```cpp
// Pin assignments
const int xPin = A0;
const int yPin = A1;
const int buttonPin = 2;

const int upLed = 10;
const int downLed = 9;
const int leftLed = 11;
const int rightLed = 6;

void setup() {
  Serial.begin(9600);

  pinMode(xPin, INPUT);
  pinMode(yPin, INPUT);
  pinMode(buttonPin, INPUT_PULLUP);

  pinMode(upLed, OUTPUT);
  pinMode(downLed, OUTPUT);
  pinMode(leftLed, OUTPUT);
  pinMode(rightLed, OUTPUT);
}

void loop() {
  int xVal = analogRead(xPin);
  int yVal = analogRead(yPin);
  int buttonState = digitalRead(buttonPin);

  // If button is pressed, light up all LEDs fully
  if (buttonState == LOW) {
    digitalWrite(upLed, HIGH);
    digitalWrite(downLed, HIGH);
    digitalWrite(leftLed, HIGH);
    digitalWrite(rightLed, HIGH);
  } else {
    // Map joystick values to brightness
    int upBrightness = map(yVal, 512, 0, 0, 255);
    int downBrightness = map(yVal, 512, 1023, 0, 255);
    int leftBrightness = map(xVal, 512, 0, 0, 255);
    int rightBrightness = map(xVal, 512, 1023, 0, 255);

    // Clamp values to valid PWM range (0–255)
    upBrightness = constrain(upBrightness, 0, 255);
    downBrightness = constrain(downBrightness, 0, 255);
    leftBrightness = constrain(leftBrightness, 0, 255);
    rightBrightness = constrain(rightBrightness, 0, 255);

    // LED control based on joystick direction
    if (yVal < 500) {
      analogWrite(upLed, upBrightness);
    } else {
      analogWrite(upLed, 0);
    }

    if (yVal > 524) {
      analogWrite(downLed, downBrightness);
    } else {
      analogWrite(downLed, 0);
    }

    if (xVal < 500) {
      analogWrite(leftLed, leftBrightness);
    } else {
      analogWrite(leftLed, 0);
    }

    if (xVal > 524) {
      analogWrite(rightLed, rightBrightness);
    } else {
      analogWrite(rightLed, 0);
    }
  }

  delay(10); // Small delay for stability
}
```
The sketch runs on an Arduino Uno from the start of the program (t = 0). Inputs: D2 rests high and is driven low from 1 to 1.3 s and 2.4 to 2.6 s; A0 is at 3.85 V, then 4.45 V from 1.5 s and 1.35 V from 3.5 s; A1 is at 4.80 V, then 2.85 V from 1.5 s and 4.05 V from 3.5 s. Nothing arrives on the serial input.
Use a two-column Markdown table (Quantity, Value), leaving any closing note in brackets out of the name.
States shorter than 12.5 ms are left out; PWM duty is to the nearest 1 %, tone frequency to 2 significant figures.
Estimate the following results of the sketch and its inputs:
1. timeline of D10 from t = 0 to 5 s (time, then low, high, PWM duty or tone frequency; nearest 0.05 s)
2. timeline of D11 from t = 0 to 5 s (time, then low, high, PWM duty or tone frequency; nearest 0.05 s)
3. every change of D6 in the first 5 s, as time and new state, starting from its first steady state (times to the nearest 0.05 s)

| Quantity | Value |
|---|---|
| timeline of D10 from t = 0 to 5 s | 0 s low; 1 s high; 1.3 s low; 2.4 s high; 2.6 s low |
| timeline of D11 from t = 0 to 5 s | 0 s low; 1 s high; 1.3 s low; 2.4 s high; 2.6 s low; 3.5 s PWM 46 % |
| every change of D6 in the first 5 s, as time and new state, starting from its first steady state | 0 s PWM 54 %; 1 s high; 1.3 s PWM 54 %; 1.5 s PWM 78 %; 2.4 s high; 2.6 s PWM 78 %; 3.5 s low |
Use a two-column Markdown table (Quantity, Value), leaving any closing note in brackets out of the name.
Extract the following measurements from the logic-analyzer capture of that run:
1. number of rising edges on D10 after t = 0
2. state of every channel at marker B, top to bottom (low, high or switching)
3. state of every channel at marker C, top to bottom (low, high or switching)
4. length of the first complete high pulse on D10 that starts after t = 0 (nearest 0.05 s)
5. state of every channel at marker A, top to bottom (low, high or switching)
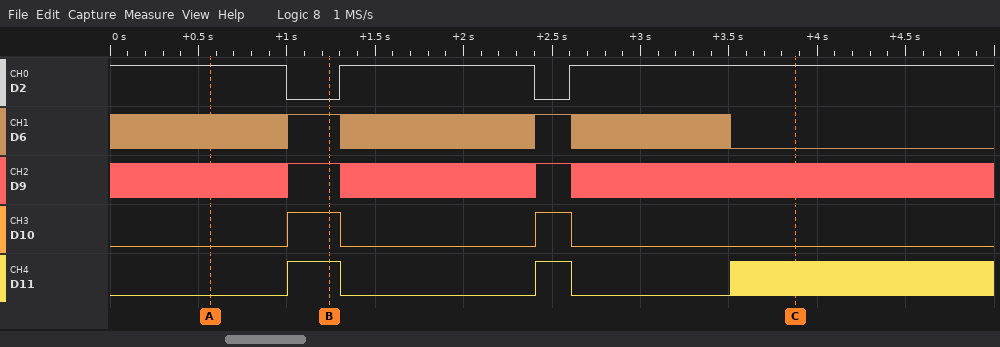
| Quantity | Value |
|---|---|
| number of rising edges on D10 after t = 0 | 2 |
| state of every channel at marker B, top to bottom | D2 low, D6 high, D9 high, D10 high, D11 high |
| state of every channel at marker C, top to bottom | D2 high, D6 low, D9 switching, D10 low, D11 switching |
| length of the first complete high pulse on D10 that starts after t = 0 | 0.30 s |
| state of every channel at marker A, top to bottom | D2 high, D6 switching, D9 switching, D10 low, D11 low |
